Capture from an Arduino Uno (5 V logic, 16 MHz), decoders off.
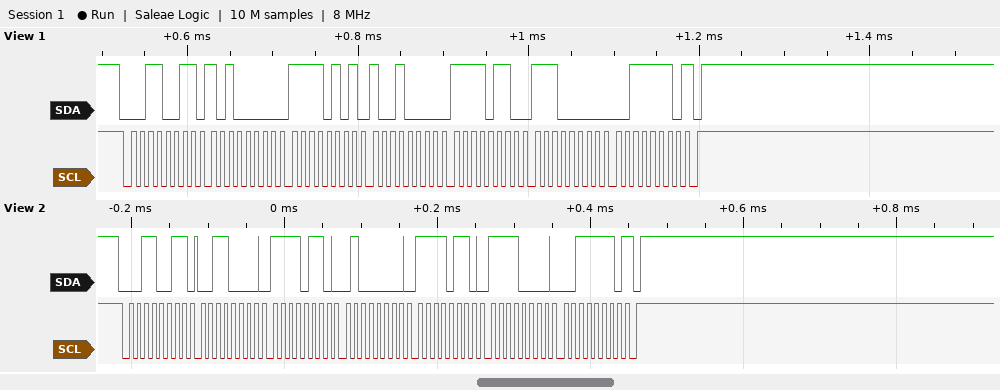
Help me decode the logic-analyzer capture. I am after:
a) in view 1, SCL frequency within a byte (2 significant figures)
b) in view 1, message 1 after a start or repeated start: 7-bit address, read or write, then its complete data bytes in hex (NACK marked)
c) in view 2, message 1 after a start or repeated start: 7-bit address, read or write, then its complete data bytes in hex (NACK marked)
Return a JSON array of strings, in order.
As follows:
["100 kHz", "0x19 read: A0 F5 90 F6 E0 3E NACK", "0x19 read: 30 F6 40 F6 F0 3E NACK"]
